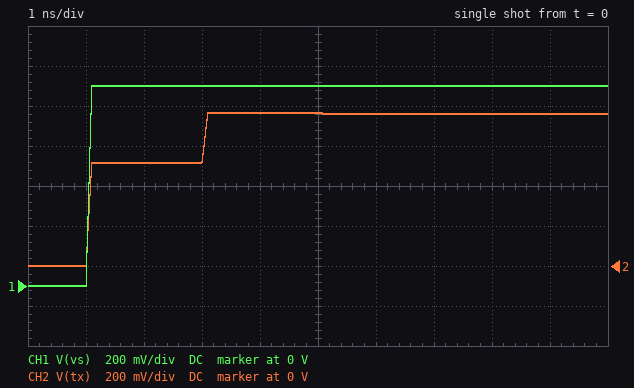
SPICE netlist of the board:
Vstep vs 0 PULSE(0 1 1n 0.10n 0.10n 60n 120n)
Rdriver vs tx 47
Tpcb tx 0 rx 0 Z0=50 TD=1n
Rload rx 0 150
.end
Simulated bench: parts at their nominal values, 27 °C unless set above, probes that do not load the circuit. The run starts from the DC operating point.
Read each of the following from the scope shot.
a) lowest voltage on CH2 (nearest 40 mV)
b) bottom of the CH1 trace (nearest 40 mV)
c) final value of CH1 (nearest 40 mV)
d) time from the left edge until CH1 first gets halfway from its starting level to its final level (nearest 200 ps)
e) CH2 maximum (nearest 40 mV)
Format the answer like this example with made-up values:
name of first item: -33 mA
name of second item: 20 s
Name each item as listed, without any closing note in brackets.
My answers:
lowest voltage on CH2: 0 V
bottom of the CH1 trace: 0 V
final value of CH1: 1.00 V
time from the left edge until CH1 first gets halfway from its starting level to its final level: 1.0 ns
CH2 maximum: 760 mV
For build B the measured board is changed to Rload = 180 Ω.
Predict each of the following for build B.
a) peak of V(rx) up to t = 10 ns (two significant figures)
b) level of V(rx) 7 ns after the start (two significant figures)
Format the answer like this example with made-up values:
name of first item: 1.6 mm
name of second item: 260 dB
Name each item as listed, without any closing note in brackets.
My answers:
peak of V(rx) up to t = 10 ns: 810 mV
level of V(rx) 7 ns after the start: 790 mV
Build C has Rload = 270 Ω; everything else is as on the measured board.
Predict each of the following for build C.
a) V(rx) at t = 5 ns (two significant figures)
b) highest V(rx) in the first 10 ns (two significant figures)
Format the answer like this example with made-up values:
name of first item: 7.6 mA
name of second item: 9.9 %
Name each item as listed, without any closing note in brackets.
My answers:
V(rx) at t = 5 ns: 850 mV
highest V(rx) in the first 10 ns: 870 mV
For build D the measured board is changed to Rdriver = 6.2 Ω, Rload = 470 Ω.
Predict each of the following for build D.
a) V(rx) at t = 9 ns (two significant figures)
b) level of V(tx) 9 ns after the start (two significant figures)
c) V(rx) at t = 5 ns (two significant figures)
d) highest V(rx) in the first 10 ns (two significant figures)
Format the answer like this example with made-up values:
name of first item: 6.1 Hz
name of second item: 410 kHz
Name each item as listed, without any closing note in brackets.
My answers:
V(rx) at t = 9 ns: 830 mV
level of V(tx) 9 ns after the start: 1.0 V
V(rx) at t = 5 ns: 600 mV
highest V(rx) in the first 10 ns: 1.6 V
